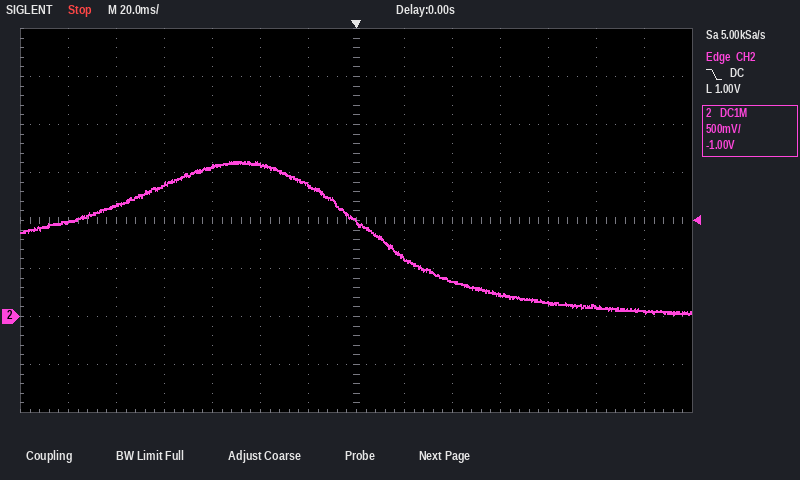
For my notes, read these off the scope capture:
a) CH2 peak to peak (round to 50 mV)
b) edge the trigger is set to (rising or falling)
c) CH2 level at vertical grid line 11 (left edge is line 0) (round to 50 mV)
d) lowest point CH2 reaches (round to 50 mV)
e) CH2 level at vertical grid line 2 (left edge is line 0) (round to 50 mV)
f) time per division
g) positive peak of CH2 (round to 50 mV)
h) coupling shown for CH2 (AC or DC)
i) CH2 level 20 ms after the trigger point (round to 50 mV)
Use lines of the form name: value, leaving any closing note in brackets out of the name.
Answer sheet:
CH2 peak to peak: 1.60 V
edge the trigger is set to: falling
CH2 level at vertical grid line 11 (left edge is line 0): 150 mV
lowest point CH2 reaches: 0 mV
CH2 level at vertical grid line 2 (left edge is line 0): 1.15 V
time per division: 20 ms
positive peak of CH2: 1.60 V
coupling shown for CH2: DC
CH2 level 20 ms after the trigger point: 600 mV
